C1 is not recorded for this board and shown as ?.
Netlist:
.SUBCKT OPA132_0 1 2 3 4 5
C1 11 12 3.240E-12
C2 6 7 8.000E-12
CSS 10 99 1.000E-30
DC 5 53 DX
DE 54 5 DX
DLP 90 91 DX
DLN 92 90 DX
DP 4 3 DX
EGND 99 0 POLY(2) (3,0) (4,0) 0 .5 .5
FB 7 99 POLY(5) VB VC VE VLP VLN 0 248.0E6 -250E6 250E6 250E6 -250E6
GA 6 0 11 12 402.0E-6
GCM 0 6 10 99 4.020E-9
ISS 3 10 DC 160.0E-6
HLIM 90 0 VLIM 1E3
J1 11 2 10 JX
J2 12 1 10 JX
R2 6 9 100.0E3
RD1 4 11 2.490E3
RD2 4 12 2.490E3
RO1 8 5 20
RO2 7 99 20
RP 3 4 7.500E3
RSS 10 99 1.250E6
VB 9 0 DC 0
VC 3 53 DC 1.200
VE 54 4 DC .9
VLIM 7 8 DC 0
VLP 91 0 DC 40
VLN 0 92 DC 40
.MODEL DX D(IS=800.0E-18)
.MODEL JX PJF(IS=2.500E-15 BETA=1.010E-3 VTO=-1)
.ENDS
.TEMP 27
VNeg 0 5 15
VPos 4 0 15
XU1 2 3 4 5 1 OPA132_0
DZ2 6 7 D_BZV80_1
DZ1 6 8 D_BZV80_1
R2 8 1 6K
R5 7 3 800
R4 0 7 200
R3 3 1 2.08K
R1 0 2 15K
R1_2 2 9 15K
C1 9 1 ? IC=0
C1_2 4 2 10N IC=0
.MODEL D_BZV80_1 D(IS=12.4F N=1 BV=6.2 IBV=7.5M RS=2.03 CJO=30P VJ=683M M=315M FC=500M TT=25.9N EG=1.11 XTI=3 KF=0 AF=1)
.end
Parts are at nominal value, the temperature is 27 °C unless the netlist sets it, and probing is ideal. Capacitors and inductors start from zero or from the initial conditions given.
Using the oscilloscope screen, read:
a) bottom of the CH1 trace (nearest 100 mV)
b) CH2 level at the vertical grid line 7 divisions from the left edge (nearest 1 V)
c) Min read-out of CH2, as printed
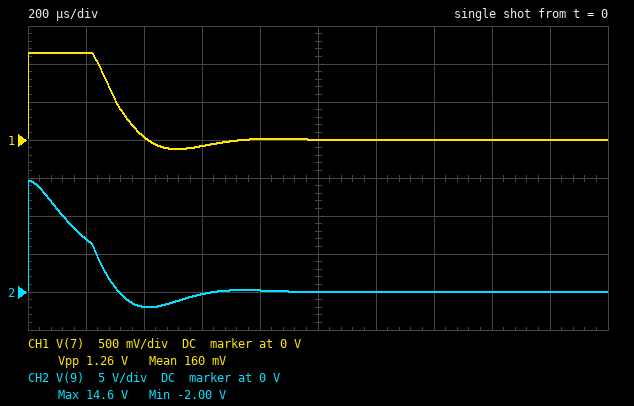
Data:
-100 mV
0 V
-2.00 V
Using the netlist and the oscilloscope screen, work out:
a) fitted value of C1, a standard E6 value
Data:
3.3 nF
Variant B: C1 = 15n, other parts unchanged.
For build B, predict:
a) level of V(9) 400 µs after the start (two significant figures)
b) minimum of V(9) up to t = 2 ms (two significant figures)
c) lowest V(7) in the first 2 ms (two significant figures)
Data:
6.9 V
-16 V
-1.2 V
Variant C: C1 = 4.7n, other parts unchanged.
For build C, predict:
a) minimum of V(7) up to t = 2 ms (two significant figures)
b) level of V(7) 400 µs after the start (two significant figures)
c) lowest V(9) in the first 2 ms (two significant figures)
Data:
-300 mV
77 mV
-4.0 V
